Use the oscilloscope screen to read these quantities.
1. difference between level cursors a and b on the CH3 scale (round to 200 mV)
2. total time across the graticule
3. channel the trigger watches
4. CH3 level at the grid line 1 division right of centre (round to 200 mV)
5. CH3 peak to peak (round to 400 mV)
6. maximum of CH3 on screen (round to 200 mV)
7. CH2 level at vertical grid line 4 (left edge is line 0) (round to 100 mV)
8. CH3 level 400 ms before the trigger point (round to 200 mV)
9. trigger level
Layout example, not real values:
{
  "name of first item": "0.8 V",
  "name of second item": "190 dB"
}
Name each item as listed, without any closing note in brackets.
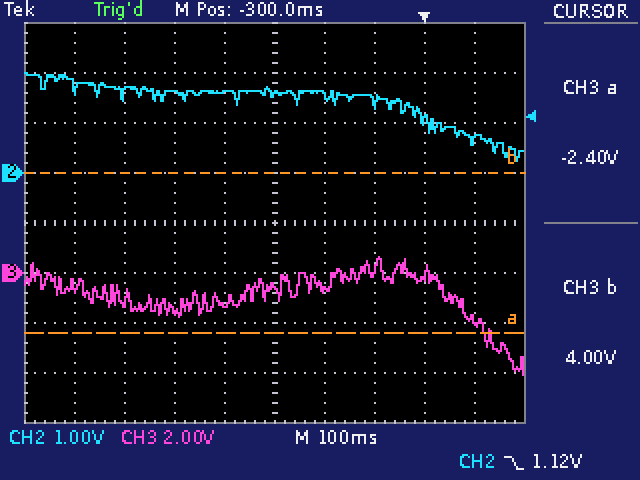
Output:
{
  "difference between level cursors a and b on the CH3 scale": "6.4 V",
  "total time across the graticule": "1 s",
  "channel the trigger watches": "CH2",
  "CH3 level at the grid line 1 division right of centre": "-600 mV",
  "CH3 peak to peak": "4.8 V",
  "maximum of CH3 on screen": "600 mV",
  "CH2 level at vertical grid line 4 (left edge is line 0)": "1.6 V",
  "CH3 level 400 ms before the trigger point": "-1.2 V",
  "trigger level": "1.12 V"
}
